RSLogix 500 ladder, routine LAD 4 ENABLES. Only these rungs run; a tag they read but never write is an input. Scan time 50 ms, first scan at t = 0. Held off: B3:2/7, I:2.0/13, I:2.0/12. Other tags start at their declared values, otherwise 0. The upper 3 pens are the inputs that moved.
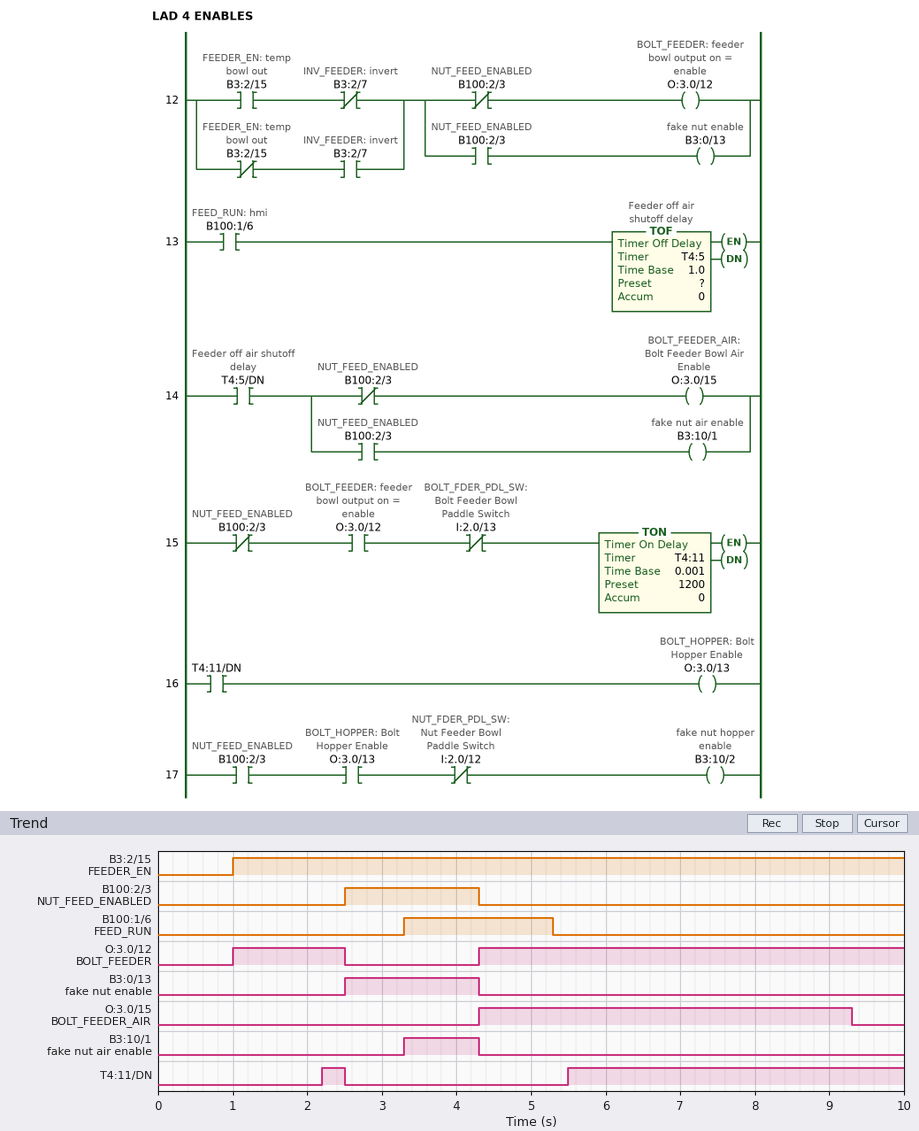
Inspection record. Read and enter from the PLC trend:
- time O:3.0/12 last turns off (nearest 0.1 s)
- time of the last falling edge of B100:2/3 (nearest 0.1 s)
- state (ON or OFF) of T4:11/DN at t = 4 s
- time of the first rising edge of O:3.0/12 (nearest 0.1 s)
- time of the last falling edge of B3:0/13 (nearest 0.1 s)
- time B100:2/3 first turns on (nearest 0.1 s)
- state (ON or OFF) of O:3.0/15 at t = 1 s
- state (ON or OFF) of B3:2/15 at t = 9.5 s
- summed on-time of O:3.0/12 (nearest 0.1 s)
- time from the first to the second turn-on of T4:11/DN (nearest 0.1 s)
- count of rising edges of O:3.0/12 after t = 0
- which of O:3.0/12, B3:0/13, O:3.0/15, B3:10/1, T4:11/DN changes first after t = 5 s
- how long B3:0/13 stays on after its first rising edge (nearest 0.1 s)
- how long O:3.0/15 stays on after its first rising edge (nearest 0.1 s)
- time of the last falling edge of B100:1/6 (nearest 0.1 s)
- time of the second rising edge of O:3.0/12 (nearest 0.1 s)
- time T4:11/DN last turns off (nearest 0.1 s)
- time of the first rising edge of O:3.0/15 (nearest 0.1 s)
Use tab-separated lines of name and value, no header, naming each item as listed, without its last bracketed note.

time O:3.0/12 last turns off	2.5 s
time of the last falling edge of B100:2/3	4.3 s
state (ON or OFF) of T4:11/DN at t = 4 s	OFF
time of the first rising edge of O:3.0/12	1.0 s
time of the last falling edge of B3:0/13	4.3 s
time B100:2/3 first turns on	2.5 s
state (ON or OFF) of O:3.0/15 at t = 1 s	OFF
state (ON or OFF) of B3:2/15 at t = 9.5 s	ON
summed on-time of O:3.0/12	7.2 s
time from the first to the second turn-on of T4:11/DN	3.3 s
count of rising edges of O:3.0/12 after t = 0	2
which of O:3.0/12, B3:0/13, O:3.0/15, B3:10/1, T4:11/DN changes first after t = 5 s	T4:11/DN
how long B3:0/13 stays on after its first rising edge	1.8 s
how long O:3.0/15 stays on after its first rising edge	5.0 s
time of the last falling edge of B100:1/6	5.3 s
time of the second rising edge of O:3.0/12	4.3 s
time T4:11/DN last turns off	2.5 s
time of the first rising edge of O:3.0/15	4.3 s
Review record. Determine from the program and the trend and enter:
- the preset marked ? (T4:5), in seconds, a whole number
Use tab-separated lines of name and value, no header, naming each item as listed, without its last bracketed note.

the preset marked ? (T4:5), in seconds, a whole number	4 s
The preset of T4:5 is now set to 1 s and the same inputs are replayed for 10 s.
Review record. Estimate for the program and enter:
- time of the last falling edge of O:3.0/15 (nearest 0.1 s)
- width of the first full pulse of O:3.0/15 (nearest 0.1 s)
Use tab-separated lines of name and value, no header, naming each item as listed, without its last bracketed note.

time of the last falling edge of O:3.0/15	6.3 s
width of the first full pulse of O:3.0/15	2.0 s
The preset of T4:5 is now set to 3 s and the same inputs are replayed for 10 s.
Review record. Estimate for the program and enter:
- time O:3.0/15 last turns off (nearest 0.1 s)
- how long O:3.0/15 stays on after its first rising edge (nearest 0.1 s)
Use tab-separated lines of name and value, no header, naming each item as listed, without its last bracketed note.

time O:3.0/15 last turns off	8.3 s
how long O:3.0/15 stays on after its first rising edge	4.0 s
